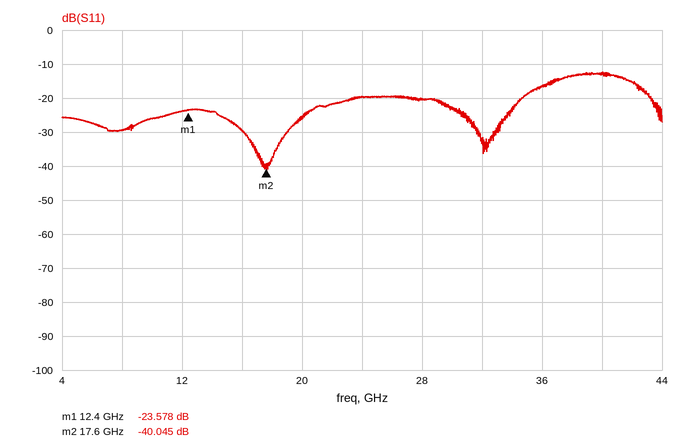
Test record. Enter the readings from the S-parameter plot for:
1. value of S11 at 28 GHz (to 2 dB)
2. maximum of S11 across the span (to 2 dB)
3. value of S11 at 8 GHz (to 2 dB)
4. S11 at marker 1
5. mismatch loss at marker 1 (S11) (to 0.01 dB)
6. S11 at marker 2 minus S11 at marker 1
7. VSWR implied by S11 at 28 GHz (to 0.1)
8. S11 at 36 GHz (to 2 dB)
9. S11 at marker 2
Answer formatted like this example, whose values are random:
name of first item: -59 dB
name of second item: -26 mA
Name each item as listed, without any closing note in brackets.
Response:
value of S11 at 28 GHz: -20 dB
maximum of S11 across the span: -12 dB
value of S11 at 8 GHz: -30 dB
S11 at marker 1: -23.578 dB
mismatch loss at marker 1 (S11): 0.02 dB
S11 at marker 2 minus S11 at marker 1: -16.467 dB
VSWR implied by S11 at 28 GHz: 1.2
S11 at 36 GHz: -16 dB
S11 at marker 2: -40.045 dB
